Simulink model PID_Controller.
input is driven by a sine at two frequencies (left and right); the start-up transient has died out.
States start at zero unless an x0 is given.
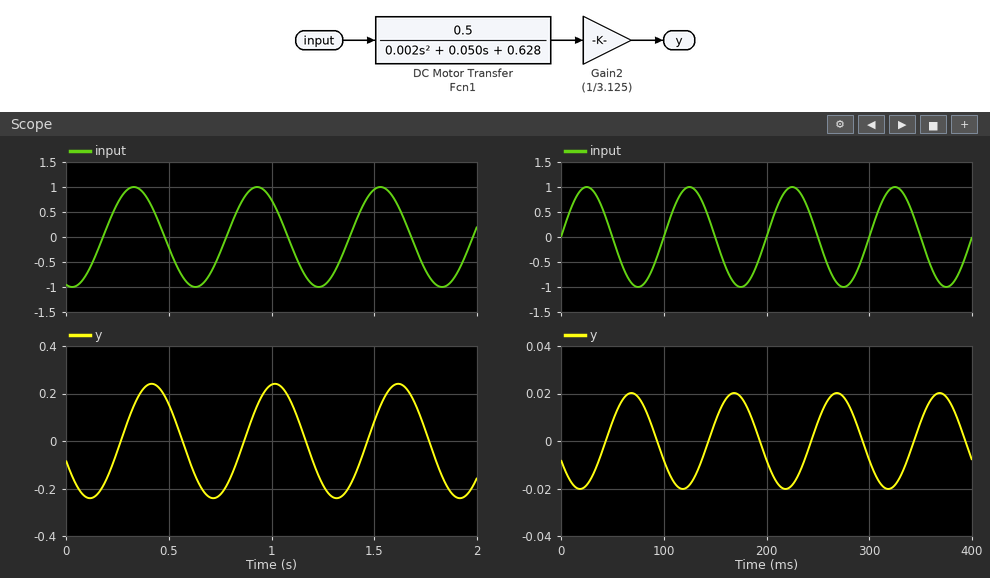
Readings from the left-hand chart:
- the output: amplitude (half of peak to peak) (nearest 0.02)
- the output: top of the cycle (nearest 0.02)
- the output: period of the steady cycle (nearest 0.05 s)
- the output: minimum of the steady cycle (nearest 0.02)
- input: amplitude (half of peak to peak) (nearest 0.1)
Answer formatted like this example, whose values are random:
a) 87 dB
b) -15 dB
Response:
a) 0.24
b) 0.24
c) 0.60 s
d) -0.24
e) 1.0
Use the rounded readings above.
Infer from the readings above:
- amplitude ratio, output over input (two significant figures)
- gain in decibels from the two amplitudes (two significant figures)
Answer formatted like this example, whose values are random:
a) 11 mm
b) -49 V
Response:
a) 0.24
b) -12 dB
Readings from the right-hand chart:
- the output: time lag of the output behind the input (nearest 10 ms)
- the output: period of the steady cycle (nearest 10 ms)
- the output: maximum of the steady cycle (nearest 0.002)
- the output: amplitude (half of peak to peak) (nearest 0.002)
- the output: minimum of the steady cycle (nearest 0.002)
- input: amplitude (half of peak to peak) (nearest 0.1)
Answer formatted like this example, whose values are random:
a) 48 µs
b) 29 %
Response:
a) 40 ms
b) 100 ms
c) 0.020
d) 0.020
e) -0.020
f) 1.0
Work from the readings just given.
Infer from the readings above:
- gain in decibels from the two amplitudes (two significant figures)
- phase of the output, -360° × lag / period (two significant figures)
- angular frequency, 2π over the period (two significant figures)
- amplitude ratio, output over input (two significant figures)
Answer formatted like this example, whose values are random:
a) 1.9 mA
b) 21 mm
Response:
a) -34 dB
b) -140°
c) 0.063 rad/ms
d) 0.020
